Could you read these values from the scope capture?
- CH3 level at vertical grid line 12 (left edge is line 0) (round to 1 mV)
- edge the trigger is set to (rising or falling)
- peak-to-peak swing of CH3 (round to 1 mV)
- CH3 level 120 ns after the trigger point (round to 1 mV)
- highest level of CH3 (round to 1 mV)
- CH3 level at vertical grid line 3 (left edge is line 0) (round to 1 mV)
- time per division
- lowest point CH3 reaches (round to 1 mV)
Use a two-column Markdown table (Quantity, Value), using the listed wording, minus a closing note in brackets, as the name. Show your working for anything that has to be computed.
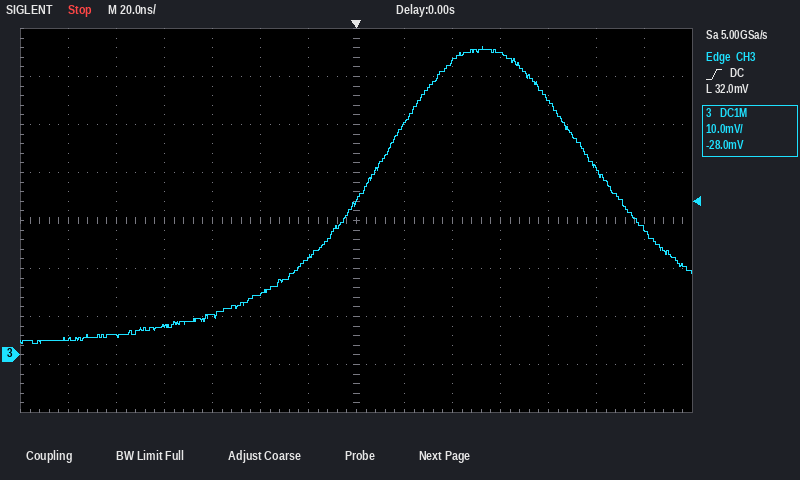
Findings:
| Quantity | Value |
|---|---|
| CH3 level at vertical grid line 12 (left edge is line 0) | 39 mV |
| edge the trigger is set to | rising |
| peak-to-peak swing of CH3 | 64 mV − (2 mV) = 62 mV |
| CH3 level 120 ns after the trigger point | 26 mV |
| highest level of CH3 | 64 mV |
| CH3 level at vertical grid line 3 (left edge is line 0) | 6 mV |
| time per division | 20 ns |
| lowest point CH3 reaches | 2 mV |
